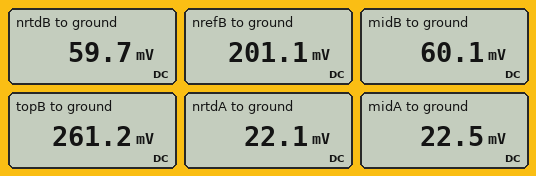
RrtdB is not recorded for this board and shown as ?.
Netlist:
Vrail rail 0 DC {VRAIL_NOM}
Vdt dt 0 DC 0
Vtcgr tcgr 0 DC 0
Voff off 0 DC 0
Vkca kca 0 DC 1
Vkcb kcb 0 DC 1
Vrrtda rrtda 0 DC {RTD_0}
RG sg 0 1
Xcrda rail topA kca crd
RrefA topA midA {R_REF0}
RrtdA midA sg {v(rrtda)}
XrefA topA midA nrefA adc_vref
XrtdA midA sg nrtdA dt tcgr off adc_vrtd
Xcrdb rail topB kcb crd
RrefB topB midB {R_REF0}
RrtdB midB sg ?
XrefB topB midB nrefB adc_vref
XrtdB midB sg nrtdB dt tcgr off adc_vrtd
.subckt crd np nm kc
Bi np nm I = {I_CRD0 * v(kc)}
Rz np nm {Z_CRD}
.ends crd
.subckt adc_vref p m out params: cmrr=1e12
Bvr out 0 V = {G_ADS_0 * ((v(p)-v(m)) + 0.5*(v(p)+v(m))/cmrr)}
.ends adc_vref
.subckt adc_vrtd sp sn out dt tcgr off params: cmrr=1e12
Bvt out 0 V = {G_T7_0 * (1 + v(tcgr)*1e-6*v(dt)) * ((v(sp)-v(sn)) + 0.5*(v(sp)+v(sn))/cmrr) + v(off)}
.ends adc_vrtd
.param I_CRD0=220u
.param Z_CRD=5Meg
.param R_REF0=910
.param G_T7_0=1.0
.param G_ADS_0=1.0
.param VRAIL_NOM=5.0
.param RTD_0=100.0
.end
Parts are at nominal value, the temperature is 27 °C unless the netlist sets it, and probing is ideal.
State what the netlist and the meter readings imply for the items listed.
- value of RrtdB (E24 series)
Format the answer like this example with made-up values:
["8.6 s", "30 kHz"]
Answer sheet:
["270 Ω"]
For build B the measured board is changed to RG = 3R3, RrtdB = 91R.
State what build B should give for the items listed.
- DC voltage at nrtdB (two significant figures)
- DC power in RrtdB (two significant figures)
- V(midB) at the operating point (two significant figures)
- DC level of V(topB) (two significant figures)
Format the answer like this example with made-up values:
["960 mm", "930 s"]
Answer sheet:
["20 mV", "4.4 µW", "22 mV", "220 mV"]
